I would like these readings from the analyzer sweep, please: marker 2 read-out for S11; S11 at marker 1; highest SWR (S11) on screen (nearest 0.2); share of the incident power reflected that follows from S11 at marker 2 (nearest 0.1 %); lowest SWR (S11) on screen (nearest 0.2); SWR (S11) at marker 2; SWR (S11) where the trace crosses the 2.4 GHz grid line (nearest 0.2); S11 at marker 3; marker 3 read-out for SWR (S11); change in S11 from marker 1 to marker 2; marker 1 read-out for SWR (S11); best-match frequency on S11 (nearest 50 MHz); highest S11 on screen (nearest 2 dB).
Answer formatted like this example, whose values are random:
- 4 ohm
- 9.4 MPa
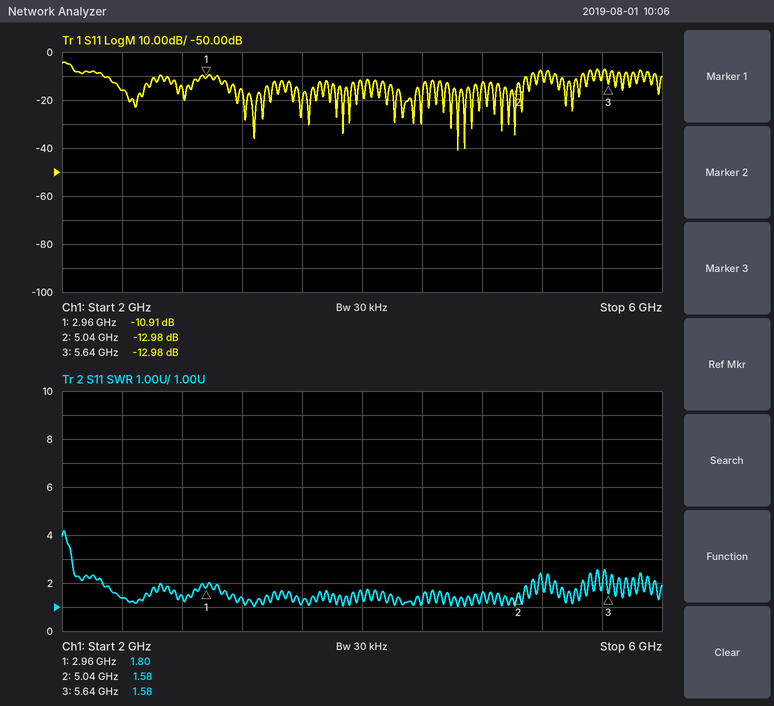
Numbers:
- -12.98 dB
- -10.91 dB
- 4.2
- 5.0 %
- 1.0
- 1.58
- 1.4
- -12.98 dB
- 1.58
- -2.07 dB
- 1.80
- 4.65 GHz
- -4 dB
